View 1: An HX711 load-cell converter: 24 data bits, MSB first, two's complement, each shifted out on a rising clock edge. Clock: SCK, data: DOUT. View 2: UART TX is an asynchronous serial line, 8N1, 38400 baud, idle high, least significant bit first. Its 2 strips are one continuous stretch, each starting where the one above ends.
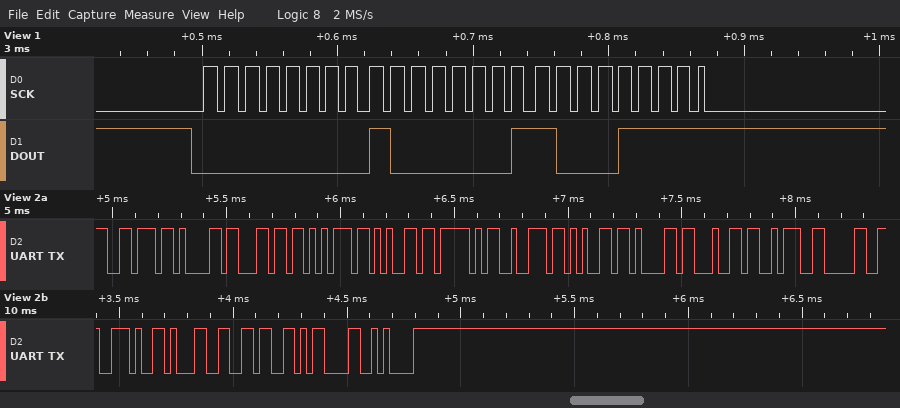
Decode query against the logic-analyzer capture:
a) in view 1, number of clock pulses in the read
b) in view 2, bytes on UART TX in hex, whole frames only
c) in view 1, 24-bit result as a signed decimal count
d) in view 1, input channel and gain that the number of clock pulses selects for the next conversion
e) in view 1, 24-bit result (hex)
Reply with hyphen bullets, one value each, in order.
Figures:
- 25
- 76 61 6C 75 65 5F 72 65 61 64 3A 30 2E 31 36 0D 0A
- 33167
- channel A, gain 128
- 0x00818F
